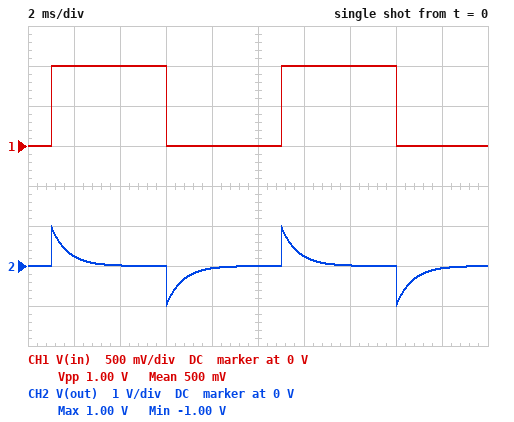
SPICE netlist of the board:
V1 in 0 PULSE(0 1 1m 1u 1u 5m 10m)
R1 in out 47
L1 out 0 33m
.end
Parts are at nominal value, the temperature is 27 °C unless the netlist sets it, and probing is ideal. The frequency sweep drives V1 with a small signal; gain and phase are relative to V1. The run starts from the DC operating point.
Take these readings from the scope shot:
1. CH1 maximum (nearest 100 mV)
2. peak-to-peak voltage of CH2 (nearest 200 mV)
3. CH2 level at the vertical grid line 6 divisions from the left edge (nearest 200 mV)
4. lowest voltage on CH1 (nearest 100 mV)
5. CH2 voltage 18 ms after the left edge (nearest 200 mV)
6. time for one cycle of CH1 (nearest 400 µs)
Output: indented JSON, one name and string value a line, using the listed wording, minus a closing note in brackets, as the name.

{
  "CH1 maximum": "1.0 V",
  "peak-to-peak voltage of CH2": "2.0 V",
  "CH2 level at the vertical grid line 6 divisions from the left edge": "200 mV",
  "lowest voltage on CH1": "0 V",
  "CH2 voltage 18 ms after the left edge": "0 V",
  "time for one cycle of CH1": "10.0 ms"
}
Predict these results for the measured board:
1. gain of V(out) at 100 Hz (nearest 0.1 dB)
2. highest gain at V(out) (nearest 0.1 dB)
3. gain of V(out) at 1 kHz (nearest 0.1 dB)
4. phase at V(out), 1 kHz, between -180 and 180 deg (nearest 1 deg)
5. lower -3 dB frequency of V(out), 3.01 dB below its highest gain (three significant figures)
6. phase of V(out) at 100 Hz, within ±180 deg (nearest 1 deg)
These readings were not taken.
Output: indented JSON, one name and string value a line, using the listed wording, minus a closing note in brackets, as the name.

{
  "gain of V(out) at 100 Hz": "-7.9 dB",
  "highest gain at V(out)": "0 dB",
  "gain of V(out) at 1 kHz": "-0.2 dB",
  "phase at V(out), 1 kHz, between -180 and 180 deg": "13 deg",
  "lower -3 dB frequency of V(out), 3.01 dB below its highest gain": "227 Hz",
  "phase of V(out) at 100 Hz, within ±180 deg": "66 deg"
}
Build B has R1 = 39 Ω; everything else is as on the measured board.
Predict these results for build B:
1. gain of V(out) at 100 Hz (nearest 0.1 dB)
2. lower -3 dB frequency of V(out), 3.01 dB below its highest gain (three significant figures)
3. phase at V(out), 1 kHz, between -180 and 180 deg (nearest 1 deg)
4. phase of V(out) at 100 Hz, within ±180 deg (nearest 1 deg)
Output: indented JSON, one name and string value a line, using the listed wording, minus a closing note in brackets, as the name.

{
  "gain of V(out) at 100 Hz": "-6.6 dB",
  "lower -3 dB frequency of V(out), 3.01 dB below its highest gain": "188 Hz",
  "phase at V(out), 1 kHz, between -180 and 180 deg": "11 deg",
  "phase of V(out) at 100 Hz, within ±180 deg": "62 deg"
}
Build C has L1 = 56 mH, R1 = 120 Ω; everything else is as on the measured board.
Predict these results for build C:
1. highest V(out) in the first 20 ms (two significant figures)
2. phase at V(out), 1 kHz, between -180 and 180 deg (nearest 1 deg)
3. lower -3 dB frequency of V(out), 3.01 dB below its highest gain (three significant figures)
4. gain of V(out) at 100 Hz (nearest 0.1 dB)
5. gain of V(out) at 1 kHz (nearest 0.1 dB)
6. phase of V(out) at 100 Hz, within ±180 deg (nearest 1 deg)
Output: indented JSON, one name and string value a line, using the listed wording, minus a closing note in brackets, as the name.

{
  "highest V(out) in the first 20 ms": "1.0 V",
  "phase at V(out), 1 kHz, between -180 and 180 deg": "19 deg",
  "lower -3 dB frequency of V(out), 3.01 dB below its highest gain": "341 Hz",
  "gain of V(out) at 100 Hz": "-11.0 dB",
  "gain of V(out) at 1 kHz": "-0.5 dB",
  "phase of V(out) at 100 Hz, within ±180 deg": "74 deg"
}
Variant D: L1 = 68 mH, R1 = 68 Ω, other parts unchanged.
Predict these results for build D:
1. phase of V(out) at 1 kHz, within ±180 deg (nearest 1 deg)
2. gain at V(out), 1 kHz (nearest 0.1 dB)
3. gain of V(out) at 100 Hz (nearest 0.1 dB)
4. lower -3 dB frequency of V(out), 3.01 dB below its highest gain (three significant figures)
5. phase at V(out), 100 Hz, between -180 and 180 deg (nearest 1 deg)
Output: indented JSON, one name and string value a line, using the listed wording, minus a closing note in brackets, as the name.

{
  "phase of V(out) at 1 kHz, within ±180 deg": "9 deg",
  "gain at V(out), 1 kHz": "-0.1 dB",
  "gain of V(out) at 100 Hz": "-5.5 dB",
  "lower -3 dB frequency of V(out), 3.01 dB below its highest gain": "159 Hz",
  "phase at V(out), 100 Hz, between -180 and 180 deg": "58 deg"
}
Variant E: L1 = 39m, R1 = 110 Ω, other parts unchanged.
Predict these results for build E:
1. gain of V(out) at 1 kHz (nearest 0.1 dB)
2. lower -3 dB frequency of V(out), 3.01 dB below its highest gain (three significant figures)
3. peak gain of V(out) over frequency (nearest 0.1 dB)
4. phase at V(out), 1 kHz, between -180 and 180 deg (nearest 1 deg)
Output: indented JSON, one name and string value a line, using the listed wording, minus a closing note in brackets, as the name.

{
  "gain of V(out) at 1 kHz": "-0.8 dB",
  "lower -3 dB frequency of V(out), 3.01 dB below its highest gain": "449 Hz",
  "peak gain of V(out) over frequency": "0 dB",
  "phase at V(out), 1 kHz, between -180 and 180 deg": "24 deg"
}
